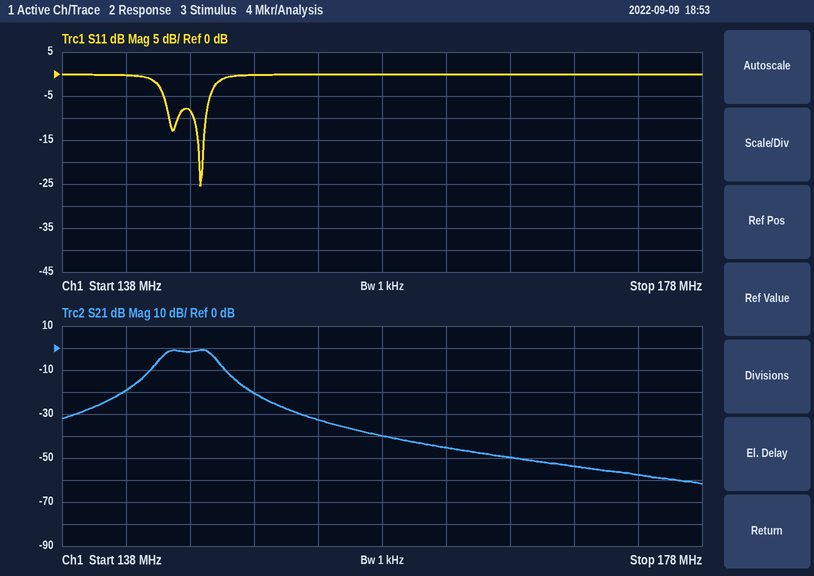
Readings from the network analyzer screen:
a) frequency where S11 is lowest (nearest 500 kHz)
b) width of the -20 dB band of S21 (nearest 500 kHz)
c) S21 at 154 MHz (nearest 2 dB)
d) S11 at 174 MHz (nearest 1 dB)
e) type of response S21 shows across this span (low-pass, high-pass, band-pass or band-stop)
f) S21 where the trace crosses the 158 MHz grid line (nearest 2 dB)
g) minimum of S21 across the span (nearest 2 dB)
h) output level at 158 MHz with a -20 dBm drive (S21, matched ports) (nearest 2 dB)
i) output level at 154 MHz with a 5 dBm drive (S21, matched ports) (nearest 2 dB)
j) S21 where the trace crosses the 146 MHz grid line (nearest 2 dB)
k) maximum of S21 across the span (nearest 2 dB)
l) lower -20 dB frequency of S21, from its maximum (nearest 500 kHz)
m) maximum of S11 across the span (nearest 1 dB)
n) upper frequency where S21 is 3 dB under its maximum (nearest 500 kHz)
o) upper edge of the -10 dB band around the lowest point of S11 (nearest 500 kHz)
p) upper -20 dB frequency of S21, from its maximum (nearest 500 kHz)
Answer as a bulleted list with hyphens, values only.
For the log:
- 146.5 MHz
- 8.5 MHz
- -32 dB
- 0 dB
- band-pass
- -40 dB
- -62 dB
- -60 dBm
- -28 dBm
- -2 dB
- 0 dB
- 141.5 MHz
- 0 dB
- 147.5 MHz
- 147.0 MHz
- 150.0 MHz
